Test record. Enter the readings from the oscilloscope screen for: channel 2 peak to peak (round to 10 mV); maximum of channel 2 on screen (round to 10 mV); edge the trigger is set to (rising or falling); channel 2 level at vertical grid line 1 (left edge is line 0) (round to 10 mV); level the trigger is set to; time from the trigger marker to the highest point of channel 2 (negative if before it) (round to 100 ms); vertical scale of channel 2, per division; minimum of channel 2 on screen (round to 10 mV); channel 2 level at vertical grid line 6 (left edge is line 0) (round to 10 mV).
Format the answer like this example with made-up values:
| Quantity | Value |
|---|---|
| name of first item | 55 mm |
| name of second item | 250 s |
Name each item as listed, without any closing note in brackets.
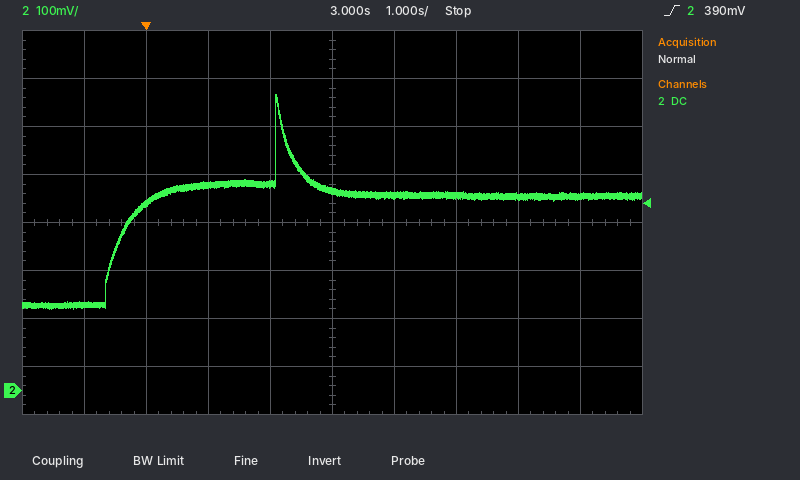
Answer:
| Quantity | Value |
|---|---|
| channel 2 peak to peak | 450 mV |
| maximum of channel 2 on screen | 620 mV |
| edge the trigger is set to | rising |
| channel 2 level at vertical grid line 1 (left edge is line 0) | 180 mV |
| level the trigger is set to | 390 mV |
| time from the trigger marker to the highest point of channel 2 (negative if before it) | +2.1 s |
| vertical scale of channel 2, per division | 100 mV |
| minimum of channel 2 on screen | 170 mV |
| channel 2 level at vertical grid line 6 (left edge is line 0) | 410 mV |
